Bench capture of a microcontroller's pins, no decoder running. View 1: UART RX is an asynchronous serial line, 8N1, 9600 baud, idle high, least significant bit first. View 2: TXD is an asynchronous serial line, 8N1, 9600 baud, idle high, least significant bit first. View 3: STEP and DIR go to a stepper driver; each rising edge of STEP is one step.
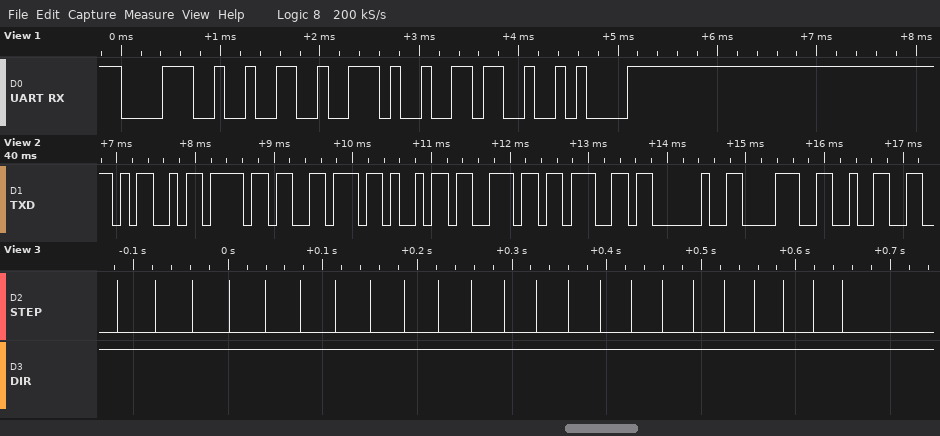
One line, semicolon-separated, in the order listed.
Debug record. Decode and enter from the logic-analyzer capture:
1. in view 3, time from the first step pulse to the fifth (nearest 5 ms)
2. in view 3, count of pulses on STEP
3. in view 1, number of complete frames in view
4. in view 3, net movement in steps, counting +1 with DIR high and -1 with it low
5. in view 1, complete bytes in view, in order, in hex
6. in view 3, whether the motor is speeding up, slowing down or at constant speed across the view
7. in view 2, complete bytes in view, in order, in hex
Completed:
155 ms; 23; 5; +23; 0x38 0x32 0x2E 0x36 0x0A; speeding up; 4D 6F 76 69 6E 67 20 38 32
